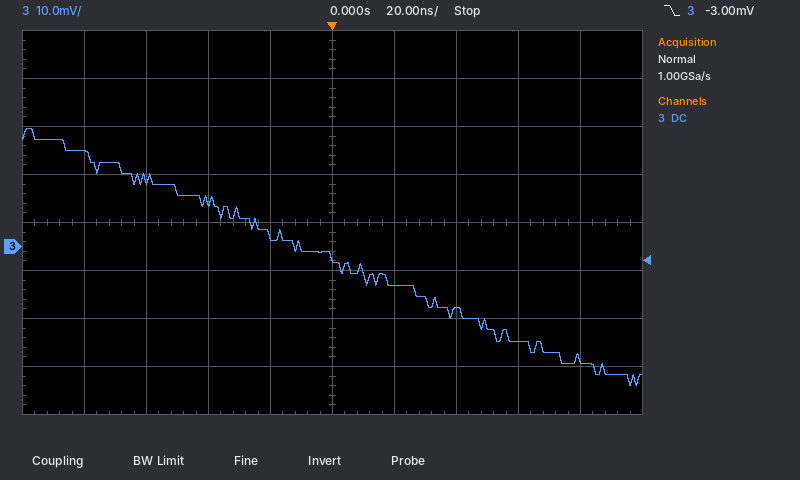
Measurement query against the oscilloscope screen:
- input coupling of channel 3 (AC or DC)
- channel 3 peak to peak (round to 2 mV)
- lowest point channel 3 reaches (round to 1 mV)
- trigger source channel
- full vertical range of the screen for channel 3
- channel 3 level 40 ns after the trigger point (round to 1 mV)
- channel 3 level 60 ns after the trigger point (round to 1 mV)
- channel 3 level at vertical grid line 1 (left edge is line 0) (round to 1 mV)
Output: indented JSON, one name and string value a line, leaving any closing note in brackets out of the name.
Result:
{
  "input coupling of channel 3": "DC",
  "channel 3 peak to peak": "54 mV",
  "lowest point channel 3 reaches": "-29 mV",
  "trigger source channel": "channel 3",
  "full vertical range of the screen for channel 3": "80 mV",
  "channel 3 level 40 ns after the trigger point": "-13 mV",
  "channel 3 level 60 ns after the trigger point": "-20 mV",
  "channel 3 level at vertical grid line 1 (left edge is line 0)": "20 mV"
}
